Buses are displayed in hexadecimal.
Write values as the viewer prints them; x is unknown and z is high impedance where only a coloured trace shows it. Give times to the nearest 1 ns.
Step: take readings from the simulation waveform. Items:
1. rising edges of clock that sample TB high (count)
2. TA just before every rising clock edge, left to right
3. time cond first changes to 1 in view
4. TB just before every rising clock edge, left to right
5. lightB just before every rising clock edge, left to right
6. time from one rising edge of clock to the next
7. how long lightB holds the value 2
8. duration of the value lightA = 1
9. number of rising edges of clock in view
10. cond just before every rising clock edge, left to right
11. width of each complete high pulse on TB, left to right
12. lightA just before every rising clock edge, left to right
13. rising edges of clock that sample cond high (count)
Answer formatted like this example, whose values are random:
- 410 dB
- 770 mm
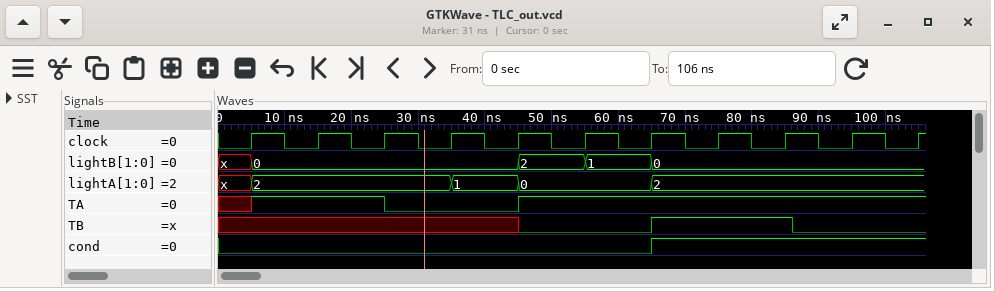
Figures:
- 2
- x 1 1 0 0 1 1 1 1 1 1
- 65 ns
- x x x x x 0 0 1 1 0 0
- x, 0, 0, 0, 0, 2, 1, 0, 0, 0, 0
- 10 ns
- 10 ns
- 10 ns
- 11
- 0 0 0 0 0 0 0 1 1 1 1
- 21 ns
- x, 2, 2, 2, 1, 0, 0, 2, 2, 2, 2
- 4
